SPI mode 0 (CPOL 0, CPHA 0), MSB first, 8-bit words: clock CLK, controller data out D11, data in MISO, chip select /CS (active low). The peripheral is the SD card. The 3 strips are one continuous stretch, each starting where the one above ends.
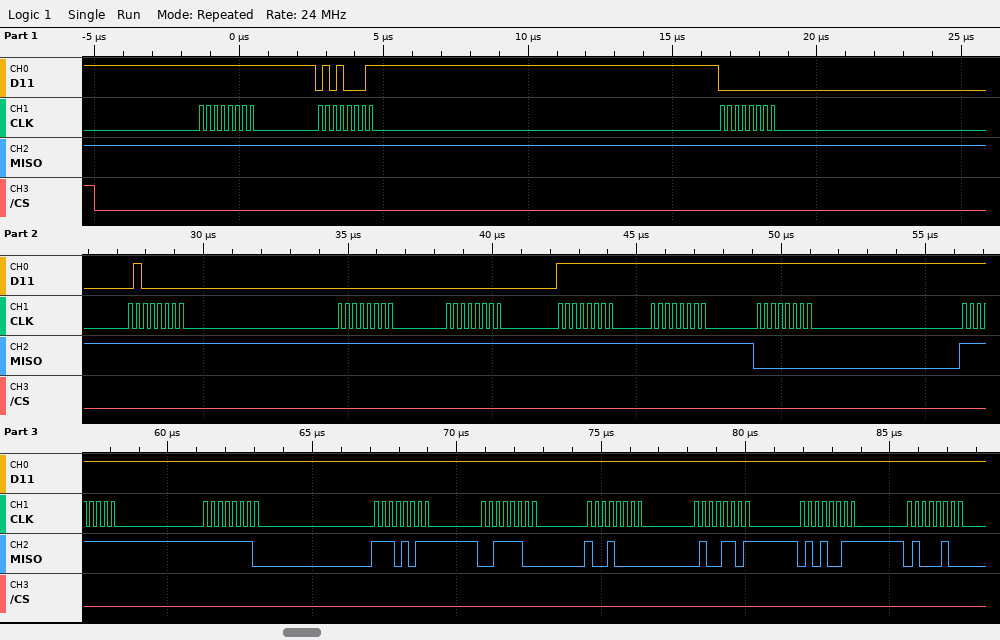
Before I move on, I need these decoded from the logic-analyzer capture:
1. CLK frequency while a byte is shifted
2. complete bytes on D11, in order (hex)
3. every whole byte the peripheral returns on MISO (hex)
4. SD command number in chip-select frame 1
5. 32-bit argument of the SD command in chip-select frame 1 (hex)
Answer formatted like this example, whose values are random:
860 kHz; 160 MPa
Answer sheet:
4 MHz; FF 51 00 40 00 00 FF FF FF FF FF FF FF FF FF FF FF; FF FF FF FF FF FF FF FF 00 FF FE EB 3C 90 4D 53 44; CMD17; 0x00400000
